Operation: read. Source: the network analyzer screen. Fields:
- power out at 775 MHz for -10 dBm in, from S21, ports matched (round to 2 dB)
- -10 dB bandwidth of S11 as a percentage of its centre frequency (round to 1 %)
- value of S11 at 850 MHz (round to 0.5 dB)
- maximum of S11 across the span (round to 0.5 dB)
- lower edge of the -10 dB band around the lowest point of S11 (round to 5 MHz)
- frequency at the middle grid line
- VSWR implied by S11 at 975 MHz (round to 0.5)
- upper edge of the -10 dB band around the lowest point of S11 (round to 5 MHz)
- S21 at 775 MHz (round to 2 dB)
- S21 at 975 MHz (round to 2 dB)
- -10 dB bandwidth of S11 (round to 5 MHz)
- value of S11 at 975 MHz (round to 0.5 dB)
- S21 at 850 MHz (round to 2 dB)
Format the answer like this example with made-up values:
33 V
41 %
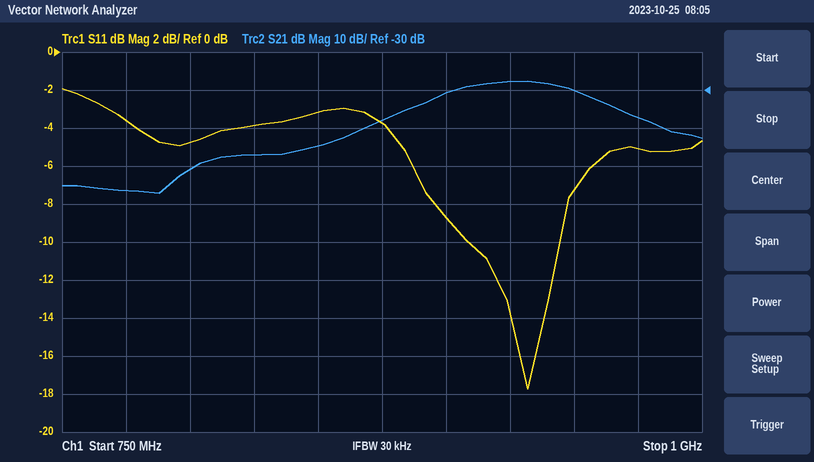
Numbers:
-66 dBm
4 %
-3.0 dB
-2.0 dB
910 MHz
875 MHz
3.5
945 MHz
-56 dB
-38 dB
35 MHz
-5.0 dB
-44 dB
